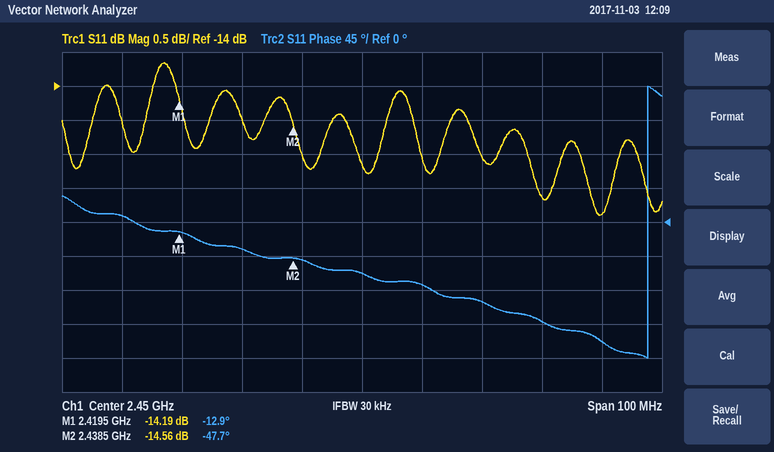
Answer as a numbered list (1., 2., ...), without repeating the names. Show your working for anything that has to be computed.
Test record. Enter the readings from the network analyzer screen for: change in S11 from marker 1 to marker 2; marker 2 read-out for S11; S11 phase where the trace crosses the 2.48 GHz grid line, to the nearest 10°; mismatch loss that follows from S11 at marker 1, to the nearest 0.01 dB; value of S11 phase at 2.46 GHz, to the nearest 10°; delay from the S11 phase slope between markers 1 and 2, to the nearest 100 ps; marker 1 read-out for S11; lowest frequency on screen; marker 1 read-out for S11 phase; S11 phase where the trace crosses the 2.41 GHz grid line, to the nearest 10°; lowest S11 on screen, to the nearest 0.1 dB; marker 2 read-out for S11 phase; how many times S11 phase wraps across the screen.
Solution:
1. -14.56 − (-14.19) = -0.37 dB
2. -14.56 dB
3. -130°
4. −10 log10(1 − 10^(-14.19/10)) ≈ 0.17 dB
5. -80°
6. −(-47.7° − (-12.9°))/(360° × 19 MHz) ≈ 5.1 ns
7. -14.19 dB
8. 2.4 GHz
9. -12.9°
10. 10°
11. -15.9 dB
12. -47.7°
13. 1
